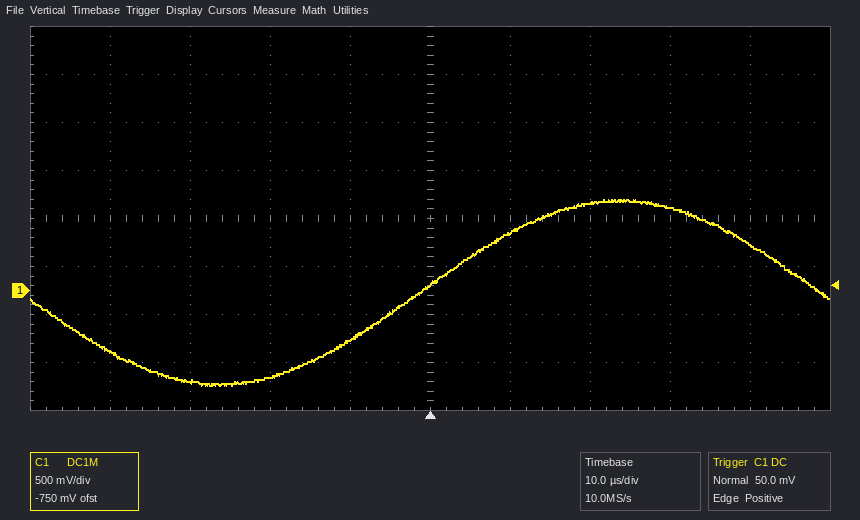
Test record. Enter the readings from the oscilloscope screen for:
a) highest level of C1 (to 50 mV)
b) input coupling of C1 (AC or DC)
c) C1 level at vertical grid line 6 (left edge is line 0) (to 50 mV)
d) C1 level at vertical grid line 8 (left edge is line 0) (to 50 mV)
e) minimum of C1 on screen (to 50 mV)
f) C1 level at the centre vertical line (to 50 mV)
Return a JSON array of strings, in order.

["950 mV", "DC", "600 mV", "850 mV", "-1.00 V", "50 mV"]
